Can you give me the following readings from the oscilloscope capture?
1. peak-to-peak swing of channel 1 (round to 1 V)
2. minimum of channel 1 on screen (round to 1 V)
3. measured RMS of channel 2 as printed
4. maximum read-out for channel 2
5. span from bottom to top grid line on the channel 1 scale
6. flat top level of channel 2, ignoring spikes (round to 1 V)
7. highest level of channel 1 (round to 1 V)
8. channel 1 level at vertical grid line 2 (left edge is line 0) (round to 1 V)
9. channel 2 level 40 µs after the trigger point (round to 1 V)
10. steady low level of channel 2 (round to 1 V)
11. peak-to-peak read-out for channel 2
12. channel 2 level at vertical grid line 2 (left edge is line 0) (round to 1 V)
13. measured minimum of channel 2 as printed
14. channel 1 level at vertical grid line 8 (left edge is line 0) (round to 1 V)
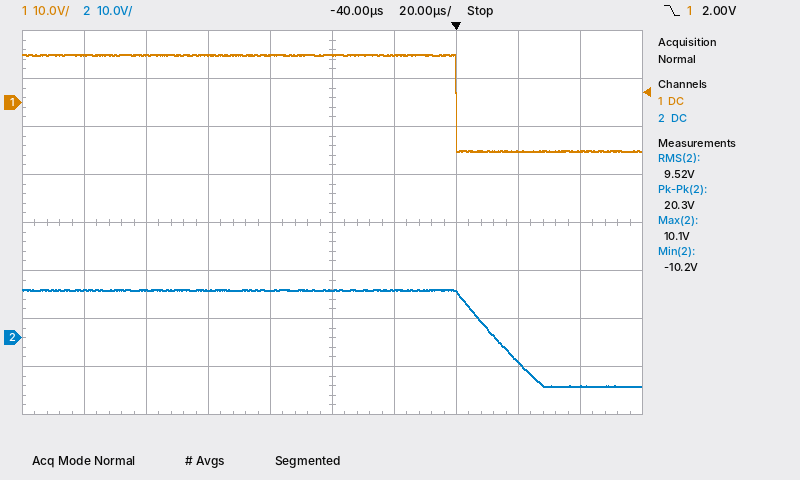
20 V
-10 V
9.52 V
10.1 V
80 V
10 V
10 V
10 V
-10 V
-10 V
20.3 V
10 V
-10.2 V
-10 V
